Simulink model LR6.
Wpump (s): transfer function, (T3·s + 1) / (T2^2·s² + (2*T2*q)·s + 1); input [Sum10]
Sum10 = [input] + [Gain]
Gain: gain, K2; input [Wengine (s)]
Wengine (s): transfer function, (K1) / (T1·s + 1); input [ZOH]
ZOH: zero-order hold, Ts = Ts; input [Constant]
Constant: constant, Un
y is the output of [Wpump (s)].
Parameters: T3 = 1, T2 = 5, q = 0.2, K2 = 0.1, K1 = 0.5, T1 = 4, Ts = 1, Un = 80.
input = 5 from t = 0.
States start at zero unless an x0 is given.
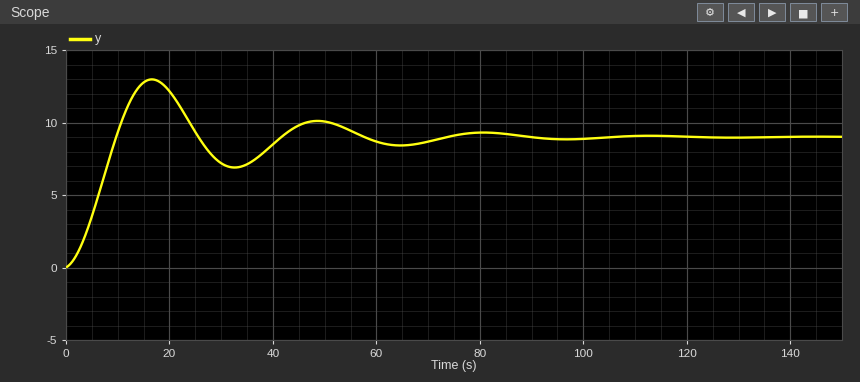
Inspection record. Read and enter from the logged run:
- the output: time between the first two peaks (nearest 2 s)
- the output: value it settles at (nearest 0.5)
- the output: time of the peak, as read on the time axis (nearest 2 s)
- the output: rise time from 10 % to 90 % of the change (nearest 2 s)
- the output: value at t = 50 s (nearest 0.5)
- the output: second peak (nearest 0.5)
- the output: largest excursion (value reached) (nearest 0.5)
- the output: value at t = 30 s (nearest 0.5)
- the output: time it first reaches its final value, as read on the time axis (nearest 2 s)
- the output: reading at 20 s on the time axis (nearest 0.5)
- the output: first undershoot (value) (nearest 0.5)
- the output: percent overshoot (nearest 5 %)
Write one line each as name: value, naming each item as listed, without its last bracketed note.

the output: time between the first two peaks: 32 s
the output: value it settles at: 9.0
the output: time of the peak, as read on the time axis: 16 s
the output: rise time from 10 % to 90 % of the change: 6 s
the output: value at t = 50 s: 10.0
the output: second peak: 10.0
the output: largest excursion (value reached): 13.0
the output: value at t = 30 s: 7.0
the output: time it first reaches its final value, as read on the time axis: 10 s
the output: reading at 20 s on the time axis: 12.0
the output: first undershoot (value): 7.0
the output: percent overshoot: 45 %
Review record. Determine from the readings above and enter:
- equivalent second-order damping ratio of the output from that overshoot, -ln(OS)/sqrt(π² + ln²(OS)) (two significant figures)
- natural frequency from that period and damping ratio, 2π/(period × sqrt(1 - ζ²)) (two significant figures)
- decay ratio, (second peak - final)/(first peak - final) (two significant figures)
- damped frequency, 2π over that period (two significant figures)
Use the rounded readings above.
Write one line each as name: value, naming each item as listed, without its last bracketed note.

equivalent second-order damping ratio of the output from that overshoot, -ln(OS)/sqrt(π² + ln²(OS)): 0.25
natural frequency from that period and damping ratio, 2π/(period × sqrt(1 - ζ²)): 0.20 rad/s
decay ratio, (second peak - final)/(first peak - final): 0.25
damped frequency, 2π over that period: 0.20 rad/s
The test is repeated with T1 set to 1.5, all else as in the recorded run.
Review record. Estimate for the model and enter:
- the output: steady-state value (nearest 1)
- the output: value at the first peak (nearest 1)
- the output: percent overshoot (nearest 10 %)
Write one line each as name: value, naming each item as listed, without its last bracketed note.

the output: steady-state value: 9
the output: value at the first peak: 14
the output: percent overshoot: 50 %
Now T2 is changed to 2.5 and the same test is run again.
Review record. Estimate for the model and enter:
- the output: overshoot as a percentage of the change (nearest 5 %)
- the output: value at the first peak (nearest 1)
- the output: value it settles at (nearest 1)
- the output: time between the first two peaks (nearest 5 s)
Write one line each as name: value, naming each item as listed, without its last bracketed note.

the output: overshoot as a percentage of the change: 35 %
the output: value at the first peak: 12
the output: value it settles at: 9
the output: time between the first two peaks: 15 s
